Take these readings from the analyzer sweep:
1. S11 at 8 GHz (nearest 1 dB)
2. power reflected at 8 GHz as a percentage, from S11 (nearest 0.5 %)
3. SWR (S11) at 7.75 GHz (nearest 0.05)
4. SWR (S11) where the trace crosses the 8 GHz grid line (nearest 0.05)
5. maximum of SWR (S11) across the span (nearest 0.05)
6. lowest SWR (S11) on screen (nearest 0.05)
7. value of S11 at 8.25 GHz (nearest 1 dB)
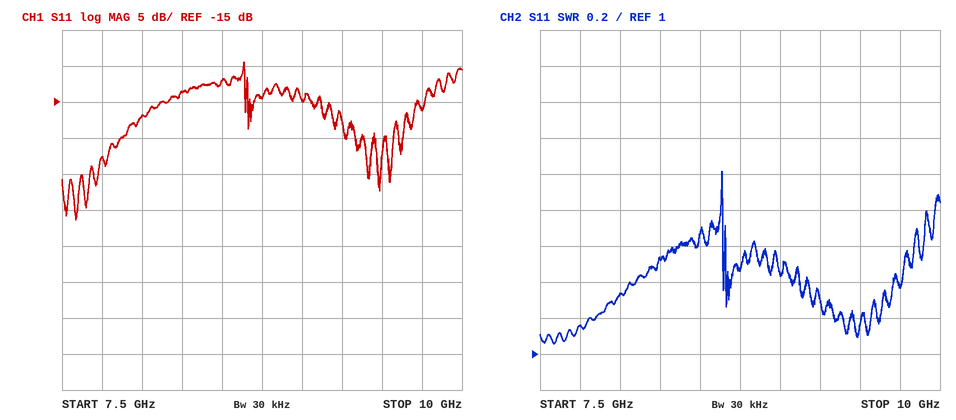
-17 dB
2.0 %
1.15
1.35
2.00
1.05
-14 dB
